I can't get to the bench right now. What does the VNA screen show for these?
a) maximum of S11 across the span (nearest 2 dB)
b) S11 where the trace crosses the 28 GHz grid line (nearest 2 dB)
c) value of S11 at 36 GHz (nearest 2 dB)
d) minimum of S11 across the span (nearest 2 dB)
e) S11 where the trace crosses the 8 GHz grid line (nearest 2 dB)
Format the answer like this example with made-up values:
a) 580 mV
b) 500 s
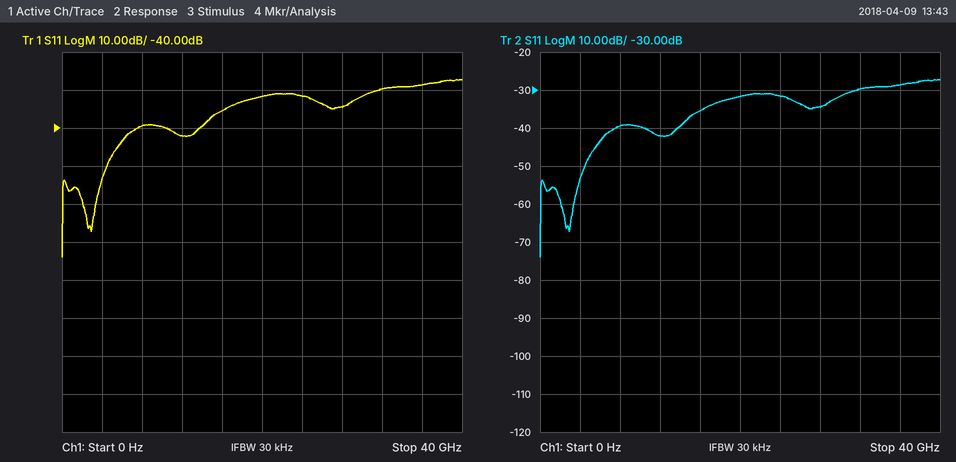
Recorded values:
a) -28 dB
b) -34 dB
c) -28 dB
d) -74 dB
e) -40 dB
